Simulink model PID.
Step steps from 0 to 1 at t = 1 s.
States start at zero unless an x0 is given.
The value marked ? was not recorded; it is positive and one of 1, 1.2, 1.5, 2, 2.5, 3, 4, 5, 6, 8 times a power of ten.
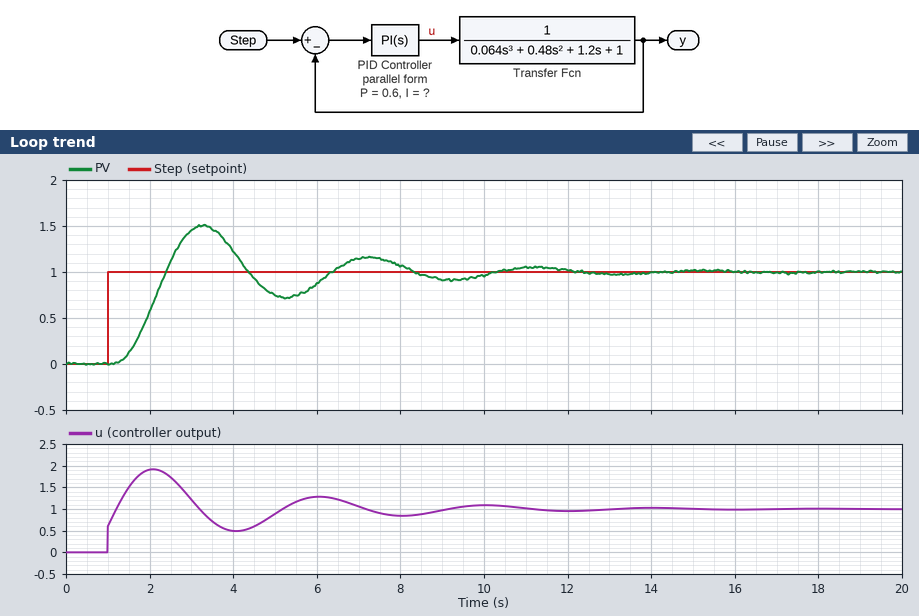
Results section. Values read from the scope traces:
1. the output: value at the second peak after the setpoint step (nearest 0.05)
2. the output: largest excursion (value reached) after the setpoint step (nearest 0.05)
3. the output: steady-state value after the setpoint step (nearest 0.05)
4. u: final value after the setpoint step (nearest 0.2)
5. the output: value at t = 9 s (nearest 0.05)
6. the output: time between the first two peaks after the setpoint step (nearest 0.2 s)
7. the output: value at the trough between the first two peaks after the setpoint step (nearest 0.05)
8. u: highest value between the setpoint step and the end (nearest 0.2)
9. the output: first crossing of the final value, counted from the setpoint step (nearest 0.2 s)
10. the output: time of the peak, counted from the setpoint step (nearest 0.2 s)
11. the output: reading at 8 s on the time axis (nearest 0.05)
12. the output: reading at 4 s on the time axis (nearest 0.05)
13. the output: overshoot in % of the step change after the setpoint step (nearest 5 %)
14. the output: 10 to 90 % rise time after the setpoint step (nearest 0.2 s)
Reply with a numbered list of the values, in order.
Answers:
1. 1.15
2. 1.50
3. 1.00
4. 1.0
5. 0.90
6. 4.0 s
7. 0.70
8. 2.0
9. 1.4 s
10. 2.2 s
11. 1.05
12. 1.25
13. 50 %
14. 0.8 s
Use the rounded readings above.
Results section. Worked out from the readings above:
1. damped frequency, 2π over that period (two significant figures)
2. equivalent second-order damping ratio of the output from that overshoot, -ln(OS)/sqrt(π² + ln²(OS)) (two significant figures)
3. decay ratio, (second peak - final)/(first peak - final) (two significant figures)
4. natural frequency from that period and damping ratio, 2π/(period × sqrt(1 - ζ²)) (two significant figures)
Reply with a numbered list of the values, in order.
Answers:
1. 1.6 rad/s
2. 0.22
3. 0.30
4. 1.6 rad/s
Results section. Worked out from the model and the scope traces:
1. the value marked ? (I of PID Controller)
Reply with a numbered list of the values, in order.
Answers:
1. 2
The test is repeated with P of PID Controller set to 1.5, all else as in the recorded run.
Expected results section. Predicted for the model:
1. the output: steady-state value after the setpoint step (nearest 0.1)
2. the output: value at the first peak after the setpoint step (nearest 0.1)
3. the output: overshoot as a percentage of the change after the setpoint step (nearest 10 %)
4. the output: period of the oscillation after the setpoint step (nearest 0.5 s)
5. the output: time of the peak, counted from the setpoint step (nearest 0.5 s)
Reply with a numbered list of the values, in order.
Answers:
1. 1.0
2. 1.3
3. 30 %
4. 3.0 s
5. 1.5 s
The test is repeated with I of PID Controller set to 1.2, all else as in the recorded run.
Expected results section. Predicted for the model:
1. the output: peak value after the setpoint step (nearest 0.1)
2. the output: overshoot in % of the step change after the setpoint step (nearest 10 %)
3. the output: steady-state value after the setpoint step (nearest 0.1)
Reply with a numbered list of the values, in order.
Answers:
1. 1.2
2. 20 %
3. 1.0
